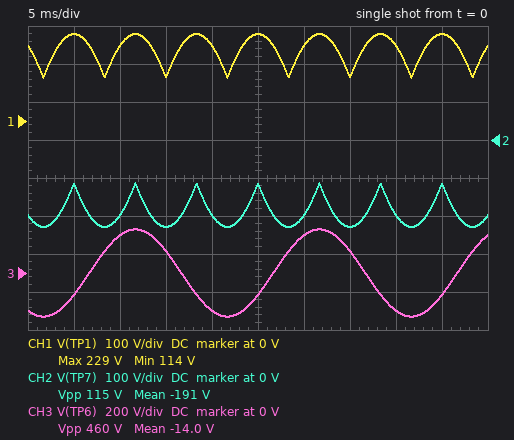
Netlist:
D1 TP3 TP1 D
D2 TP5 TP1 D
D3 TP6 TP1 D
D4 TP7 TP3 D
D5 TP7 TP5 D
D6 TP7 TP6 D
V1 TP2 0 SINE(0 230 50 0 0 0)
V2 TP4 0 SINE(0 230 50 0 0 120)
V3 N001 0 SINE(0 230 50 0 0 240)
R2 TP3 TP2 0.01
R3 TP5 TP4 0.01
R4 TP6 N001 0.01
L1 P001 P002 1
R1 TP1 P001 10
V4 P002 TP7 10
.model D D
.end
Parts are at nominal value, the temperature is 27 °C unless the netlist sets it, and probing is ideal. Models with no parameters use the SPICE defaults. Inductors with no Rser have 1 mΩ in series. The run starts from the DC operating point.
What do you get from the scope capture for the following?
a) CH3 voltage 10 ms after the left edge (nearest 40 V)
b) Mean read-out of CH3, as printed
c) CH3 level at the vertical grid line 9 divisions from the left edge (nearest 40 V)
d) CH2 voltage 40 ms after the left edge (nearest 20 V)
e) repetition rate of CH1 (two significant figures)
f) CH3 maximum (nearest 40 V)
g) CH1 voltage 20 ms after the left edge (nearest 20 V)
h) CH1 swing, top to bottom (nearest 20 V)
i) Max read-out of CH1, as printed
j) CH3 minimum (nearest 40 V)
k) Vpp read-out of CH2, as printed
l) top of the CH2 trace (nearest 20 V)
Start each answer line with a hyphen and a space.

- 200 V
- -14.0 V
- -120 V
- -200 V
- 150 Hz
- 240 V
- 200 V
- 120 V
- 229 V
- -240 V
- 115 V
- -120 V
